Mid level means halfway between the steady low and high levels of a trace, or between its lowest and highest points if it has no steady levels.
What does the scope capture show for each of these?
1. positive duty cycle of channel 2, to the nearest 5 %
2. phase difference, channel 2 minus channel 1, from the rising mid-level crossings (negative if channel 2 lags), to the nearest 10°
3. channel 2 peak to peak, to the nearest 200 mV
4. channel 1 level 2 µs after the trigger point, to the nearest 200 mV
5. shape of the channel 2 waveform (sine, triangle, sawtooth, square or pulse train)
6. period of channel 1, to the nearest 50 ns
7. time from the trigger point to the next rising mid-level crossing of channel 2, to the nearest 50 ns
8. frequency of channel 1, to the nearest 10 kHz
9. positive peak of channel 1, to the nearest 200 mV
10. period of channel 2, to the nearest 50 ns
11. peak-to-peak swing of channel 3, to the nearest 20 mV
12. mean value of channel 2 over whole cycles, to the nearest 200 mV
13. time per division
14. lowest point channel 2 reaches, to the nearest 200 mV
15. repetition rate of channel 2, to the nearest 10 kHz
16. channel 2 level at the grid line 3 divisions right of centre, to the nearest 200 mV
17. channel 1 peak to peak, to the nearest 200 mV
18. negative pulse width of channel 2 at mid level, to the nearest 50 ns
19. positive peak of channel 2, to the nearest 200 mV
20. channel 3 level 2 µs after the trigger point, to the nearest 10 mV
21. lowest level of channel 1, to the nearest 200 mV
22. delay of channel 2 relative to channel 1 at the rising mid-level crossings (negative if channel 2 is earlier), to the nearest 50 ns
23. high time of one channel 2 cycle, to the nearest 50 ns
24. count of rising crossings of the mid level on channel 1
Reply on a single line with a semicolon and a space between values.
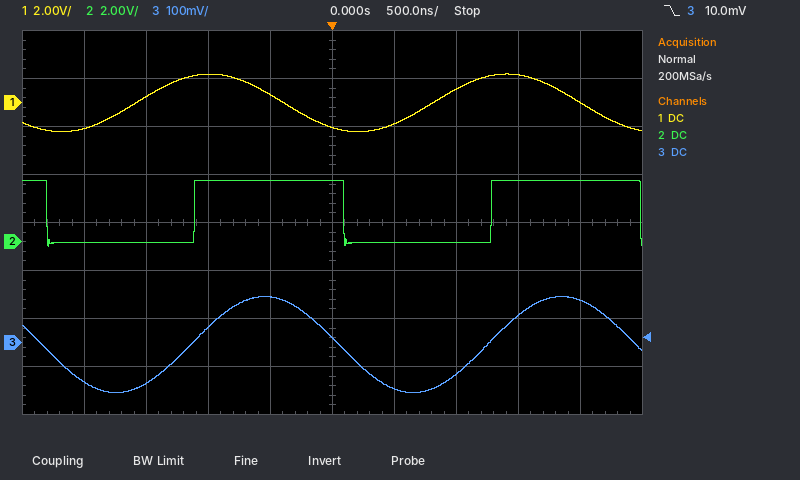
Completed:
50 %; -70°; 2.8 V; 0.0 V; square; 2.40 µs; 1.30 µs; 420 kHz; 1.2 V; 2.40 µs; 200 mV; 1.2 V; 500 ns; -200 mV; 420 kHz; 2.6 V; 2.4 V; 1.20 µs; 2.6 V; 90 mV; -1.2 V; +450 ns; 1.20 µs; 2
